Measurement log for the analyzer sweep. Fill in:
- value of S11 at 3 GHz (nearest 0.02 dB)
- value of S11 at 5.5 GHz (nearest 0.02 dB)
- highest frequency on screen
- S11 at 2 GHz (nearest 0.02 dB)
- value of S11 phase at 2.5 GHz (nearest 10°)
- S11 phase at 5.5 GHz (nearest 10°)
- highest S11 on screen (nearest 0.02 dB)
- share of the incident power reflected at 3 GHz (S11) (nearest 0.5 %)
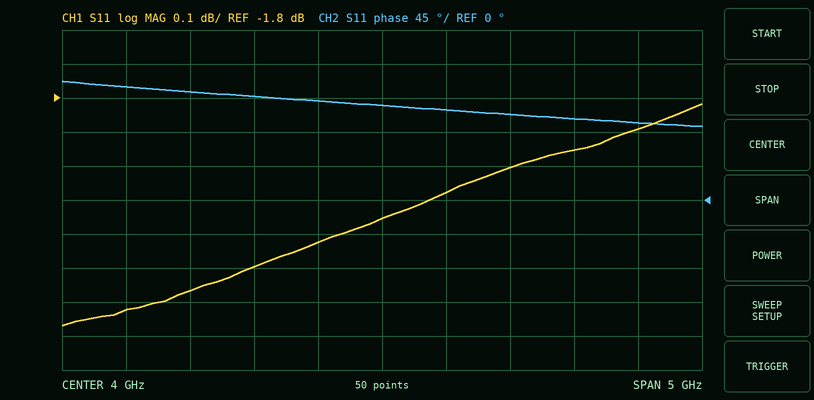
-2.30 dB
-1.96 dB
6.5 GHz
-2.42 dB
140°
110°
-1.82 dB
59.0 %
